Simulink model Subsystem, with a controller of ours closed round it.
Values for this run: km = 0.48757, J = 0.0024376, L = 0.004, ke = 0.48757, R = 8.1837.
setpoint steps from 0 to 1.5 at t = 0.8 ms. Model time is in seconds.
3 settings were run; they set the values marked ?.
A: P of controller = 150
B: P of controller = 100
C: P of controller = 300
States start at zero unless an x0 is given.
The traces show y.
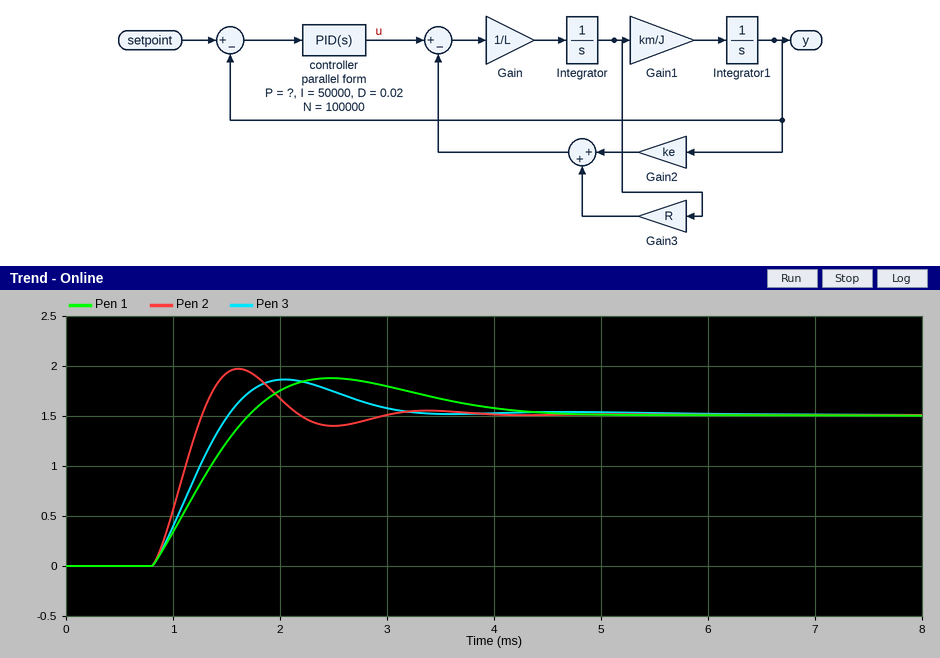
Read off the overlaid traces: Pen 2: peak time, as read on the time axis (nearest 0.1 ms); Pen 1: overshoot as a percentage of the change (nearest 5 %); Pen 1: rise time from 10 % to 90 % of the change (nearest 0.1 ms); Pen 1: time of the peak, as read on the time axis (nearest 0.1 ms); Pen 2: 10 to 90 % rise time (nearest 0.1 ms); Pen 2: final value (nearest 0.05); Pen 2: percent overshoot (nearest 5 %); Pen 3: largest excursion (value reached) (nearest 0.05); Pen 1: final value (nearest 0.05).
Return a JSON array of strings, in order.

["1.6 ms", "25 %", "0.7 ms", "2.5 ms", "0.3 ms", "1.50", "30 %", "1.85", "1.50"]
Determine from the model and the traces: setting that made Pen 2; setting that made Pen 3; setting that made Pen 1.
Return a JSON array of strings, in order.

["C", "A", "B"]
